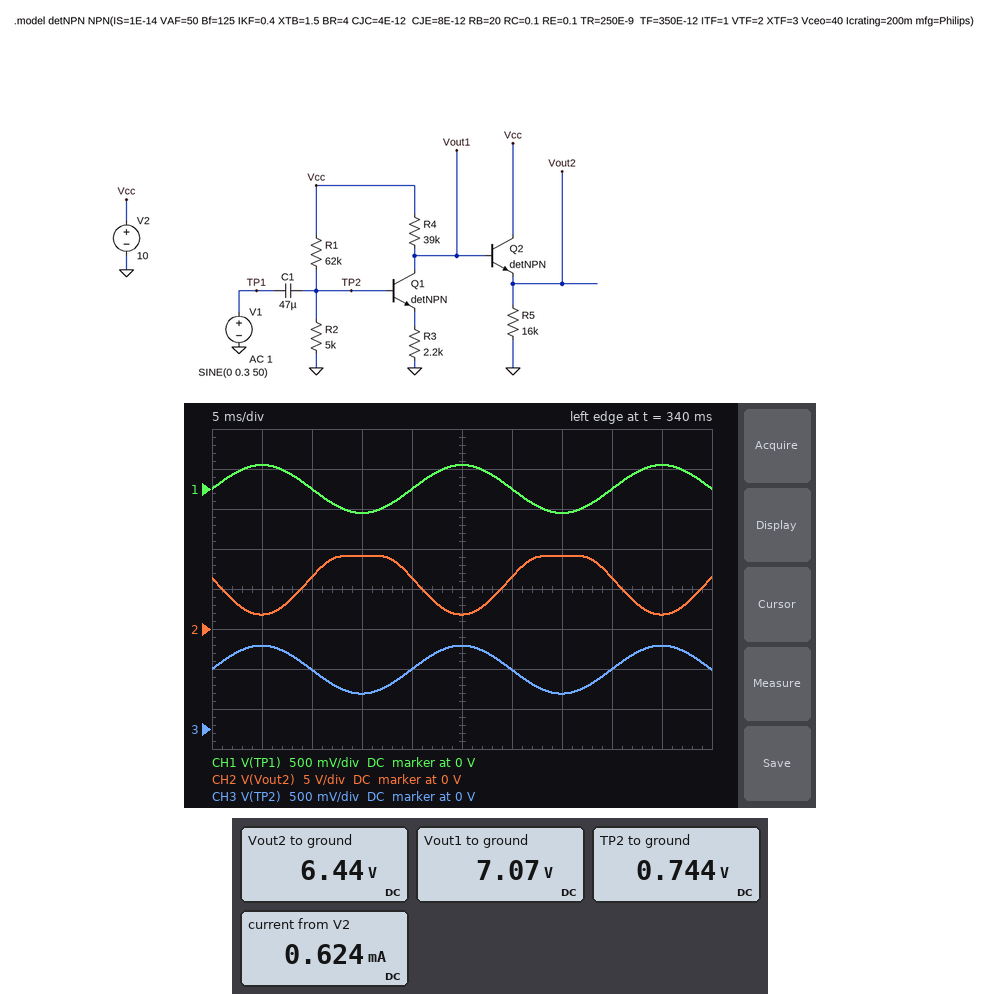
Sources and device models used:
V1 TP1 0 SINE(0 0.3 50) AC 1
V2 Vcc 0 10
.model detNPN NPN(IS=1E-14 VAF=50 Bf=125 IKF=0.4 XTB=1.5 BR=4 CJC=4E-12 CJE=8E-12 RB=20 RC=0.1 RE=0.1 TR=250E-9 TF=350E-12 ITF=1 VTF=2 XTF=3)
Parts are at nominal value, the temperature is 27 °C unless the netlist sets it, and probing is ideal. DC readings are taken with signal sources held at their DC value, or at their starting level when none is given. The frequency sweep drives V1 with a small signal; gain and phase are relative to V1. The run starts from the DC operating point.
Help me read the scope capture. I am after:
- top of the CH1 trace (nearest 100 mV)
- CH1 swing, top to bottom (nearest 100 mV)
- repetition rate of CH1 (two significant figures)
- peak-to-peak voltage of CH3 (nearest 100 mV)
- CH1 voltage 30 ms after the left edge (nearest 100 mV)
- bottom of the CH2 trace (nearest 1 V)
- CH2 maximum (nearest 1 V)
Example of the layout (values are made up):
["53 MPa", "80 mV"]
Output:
["300 mV", "600 mV", "50 Hz", "600 mV", "0 V", "2 V", "9 V"]
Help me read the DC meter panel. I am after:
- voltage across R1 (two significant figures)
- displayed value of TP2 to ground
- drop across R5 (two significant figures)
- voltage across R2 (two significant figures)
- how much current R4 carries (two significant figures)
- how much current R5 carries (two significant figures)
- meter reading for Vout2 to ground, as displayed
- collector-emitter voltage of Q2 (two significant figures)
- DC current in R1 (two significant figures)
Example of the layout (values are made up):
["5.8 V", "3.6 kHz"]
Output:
["9.3 V", "0.744 V", "6.4 V", "740 mV", "75 µA", "400 µA", "6.44 V", "3.6 V", "150 µA"]
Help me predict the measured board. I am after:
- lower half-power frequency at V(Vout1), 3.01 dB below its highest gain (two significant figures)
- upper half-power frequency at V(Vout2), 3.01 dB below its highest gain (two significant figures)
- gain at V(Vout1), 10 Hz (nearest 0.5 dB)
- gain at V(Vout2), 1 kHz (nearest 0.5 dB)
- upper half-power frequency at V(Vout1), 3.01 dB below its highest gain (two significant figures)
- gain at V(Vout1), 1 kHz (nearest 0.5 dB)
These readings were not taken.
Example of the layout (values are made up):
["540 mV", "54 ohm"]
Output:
["740 mHz", "960 kHz", "23.5 dB", "23.5 dB", "960 kHz", "23.5 dB"]
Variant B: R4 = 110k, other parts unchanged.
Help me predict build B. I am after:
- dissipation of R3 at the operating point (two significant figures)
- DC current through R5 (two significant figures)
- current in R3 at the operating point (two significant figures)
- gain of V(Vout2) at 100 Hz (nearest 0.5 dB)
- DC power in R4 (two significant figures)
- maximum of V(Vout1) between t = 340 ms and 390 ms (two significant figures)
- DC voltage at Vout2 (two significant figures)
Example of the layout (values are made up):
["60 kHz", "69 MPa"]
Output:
["11 µW", "95 µA", "72 µA", "32.0 dB", "570 µW", "9.5 V", "1.5 V"]
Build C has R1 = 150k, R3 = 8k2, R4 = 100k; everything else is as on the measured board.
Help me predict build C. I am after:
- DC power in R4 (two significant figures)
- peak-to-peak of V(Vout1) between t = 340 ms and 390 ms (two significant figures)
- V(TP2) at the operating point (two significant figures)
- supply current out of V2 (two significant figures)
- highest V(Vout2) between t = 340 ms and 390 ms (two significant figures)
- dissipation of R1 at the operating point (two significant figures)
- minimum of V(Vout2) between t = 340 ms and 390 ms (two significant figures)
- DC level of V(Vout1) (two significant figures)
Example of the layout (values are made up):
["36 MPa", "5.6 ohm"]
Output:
["1.9 µW", "1.0 V", "320 mV", "620 µA", "8.9 V", "620 µW", "7.9 V", "9.6 V"]
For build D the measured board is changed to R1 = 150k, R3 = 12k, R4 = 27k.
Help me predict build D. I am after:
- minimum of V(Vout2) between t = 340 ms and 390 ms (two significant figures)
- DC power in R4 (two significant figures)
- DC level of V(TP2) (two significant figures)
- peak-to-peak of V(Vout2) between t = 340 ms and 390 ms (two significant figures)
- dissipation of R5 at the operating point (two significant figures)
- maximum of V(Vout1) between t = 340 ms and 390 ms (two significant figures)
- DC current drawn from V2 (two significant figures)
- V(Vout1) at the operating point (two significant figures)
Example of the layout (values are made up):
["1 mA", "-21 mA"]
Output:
["9.0 V", "570 nW", "320 mV", "210 mV", "5.3 mW", "9.9 V", "640 µA", "9.9 V"]
